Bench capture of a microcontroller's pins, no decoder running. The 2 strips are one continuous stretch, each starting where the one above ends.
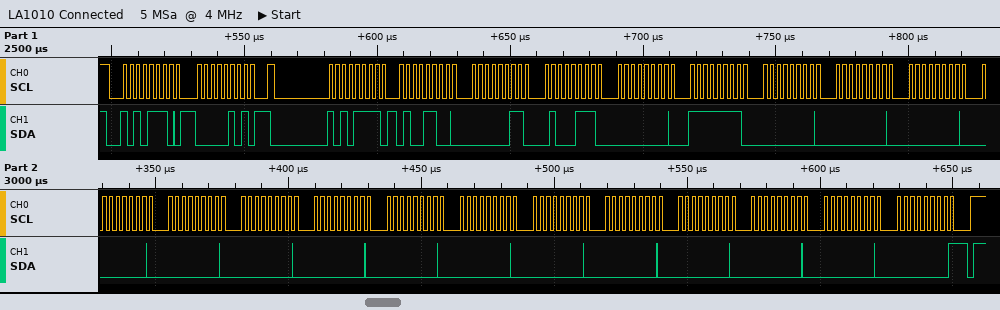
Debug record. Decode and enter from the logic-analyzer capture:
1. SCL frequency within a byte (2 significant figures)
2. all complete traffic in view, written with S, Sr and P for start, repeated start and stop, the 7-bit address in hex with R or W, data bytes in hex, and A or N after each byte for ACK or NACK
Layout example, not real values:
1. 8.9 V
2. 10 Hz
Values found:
1. 400 kHz
2. S 57W A 05 A Sr 57R A 4C A 03 A 47 A 00 A FF A 00 A 00 A 00 A 00 A 00 A 00 A 00 A 00 A 00 A 00 A 00 A 00 A 00 A 00 A 00 N P
